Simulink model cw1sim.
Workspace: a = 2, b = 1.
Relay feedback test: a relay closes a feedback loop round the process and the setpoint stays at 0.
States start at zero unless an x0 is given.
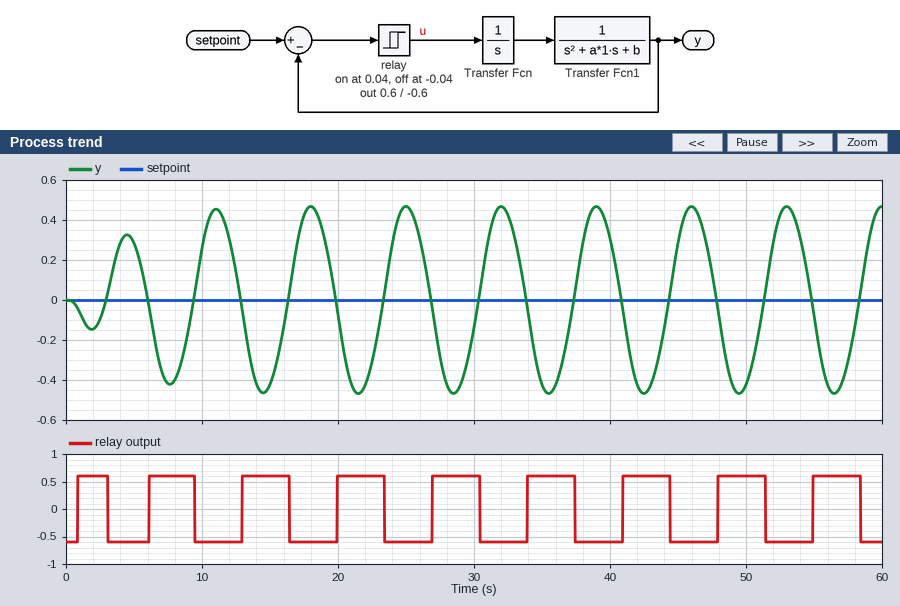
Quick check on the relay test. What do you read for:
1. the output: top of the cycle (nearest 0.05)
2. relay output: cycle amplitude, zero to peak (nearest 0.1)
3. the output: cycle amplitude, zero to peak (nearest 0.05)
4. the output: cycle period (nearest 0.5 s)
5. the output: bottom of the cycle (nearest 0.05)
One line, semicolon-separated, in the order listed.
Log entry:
0.45; 0.6; 0.45; 7.0 s; -0.45
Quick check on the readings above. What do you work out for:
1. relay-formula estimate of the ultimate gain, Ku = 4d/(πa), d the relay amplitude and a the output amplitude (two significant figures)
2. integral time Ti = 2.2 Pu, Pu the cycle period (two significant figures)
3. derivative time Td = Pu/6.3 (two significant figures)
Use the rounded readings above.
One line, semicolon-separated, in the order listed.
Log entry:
1.7; 15 s; 1.1 s
